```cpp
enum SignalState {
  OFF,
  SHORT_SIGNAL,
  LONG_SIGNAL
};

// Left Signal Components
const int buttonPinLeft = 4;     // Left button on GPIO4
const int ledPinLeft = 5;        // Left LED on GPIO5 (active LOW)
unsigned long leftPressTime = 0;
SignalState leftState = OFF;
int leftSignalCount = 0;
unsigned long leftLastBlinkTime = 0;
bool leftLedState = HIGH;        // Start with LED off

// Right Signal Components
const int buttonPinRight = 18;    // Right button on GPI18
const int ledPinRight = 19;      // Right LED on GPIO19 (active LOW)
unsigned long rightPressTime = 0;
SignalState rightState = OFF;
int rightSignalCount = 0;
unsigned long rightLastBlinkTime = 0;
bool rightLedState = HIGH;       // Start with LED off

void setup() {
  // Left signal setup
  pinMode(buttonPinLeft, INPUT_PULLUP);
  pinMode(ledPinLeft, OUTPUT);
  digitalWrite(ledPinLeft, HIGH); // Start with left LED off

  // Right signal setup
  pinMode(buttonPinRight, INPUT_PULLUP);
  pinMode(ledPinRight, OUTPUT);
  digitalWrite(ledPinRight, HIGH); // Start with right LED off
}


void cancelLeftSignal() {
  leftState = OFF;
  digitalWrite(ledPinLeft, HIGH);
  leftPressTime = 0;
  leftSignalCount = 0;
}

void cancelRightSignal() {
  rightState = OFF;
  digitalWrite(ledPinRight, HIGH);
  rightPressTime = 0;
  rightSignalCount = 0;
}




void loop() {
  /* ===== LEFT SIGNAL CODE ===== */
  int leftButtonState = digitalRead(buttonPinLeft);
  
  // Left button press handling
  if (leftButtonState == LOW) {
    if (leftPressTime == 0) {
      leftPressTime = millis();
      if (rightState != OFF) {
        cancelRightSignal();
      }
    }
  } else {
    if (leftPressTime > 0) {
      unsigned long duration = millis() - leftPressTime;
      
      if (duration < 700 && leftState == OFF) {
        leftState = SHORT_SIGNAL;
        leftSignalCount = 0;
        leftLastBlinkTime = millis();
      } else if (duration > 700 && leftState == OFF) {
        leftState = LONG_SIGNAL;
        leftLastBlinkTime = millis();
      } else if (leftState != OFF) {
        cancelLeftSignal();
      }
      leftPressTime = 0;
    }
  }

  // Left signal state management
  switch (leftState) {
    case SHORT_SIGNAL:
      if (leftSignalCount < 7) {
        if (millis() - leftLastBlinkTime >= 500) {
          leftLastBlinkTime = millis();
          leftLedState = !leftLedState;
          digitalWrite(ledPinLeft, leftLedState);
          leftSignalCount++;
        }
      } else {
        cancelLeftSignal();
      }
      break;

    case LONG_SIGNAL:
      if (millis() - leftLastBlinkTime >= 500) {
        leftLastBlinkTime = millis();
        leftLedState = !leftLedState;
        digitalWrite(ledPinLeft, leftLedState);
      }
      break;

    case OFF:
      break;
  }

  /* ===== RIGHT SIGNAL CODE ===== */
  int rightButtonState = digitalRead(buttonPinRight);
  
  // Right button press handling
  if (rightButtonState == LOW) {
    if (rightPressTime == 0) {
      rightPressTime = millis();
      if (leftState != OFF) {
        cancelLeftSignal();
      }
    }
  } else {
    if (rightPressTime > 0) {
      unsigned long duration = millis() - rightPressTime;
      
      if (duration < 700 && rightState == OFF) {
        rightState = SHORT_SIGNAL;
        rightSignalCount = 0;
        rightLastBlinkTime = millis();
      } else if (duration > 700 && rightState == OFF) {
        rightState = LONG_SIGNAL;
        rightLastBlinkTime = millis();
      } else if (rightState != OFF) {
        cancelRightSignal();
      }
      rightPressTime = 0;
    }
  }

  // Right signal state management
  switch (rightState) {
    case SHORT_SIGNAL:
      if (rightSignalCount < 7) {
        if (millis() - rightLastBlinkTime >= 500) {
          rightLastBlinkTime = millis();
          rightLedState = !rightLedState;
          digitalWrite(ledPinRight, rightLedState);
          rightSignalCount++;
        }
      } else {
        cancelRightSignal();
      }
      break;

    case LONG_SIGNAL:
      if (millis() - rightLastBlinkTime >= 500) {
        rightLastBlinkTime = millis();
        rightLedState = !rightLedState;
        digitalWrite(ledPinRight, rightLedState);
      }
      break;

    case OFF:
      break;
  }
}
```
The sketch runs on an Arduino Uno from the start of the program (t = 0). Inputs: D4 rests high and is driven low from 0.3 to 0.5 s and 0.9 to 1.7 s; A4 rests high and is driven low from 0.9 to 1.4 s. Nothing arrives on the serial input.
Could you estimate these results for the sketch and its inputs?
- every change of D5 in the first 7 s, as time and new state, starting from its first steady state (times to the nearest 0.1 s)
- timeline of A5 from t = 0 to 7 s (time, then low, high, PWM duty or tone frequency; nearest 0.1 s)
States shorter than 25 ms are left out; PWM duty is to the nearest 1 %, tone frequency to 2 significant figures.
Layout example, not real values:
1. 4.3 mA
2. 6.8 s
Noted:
1. 0 s high; 2.2 s low; 2.7 s high; 3.2 s low; 3.7 s high; 4.2 s low; 4.7 s high; 5.2 s low; 5.7 s high; 6.2 s low; 6.7 s high
2. 0 s high; 1.9 s low; 2.4 s high; 2.9 s low; 3.4 s high; 3.9 s low; 4.4 s high
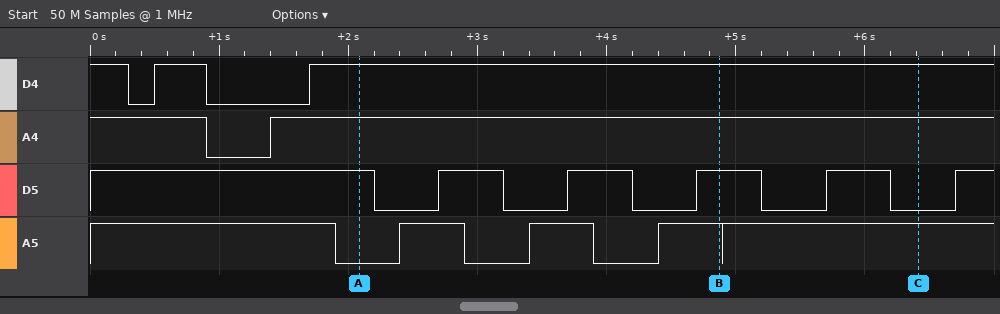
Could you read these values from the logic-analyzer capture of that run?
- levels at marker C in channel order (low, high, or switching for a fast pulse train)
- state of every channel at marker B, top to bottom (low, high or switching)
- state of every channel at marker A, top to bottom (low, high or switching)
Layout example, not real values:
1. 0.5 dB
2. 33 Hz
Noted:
1. D4 high, A4 high, D5 low, A5 high
2. D4 high, A4 high, D5 high, A5 high
3. D4 high, A4 high, D5 high, A5 low
